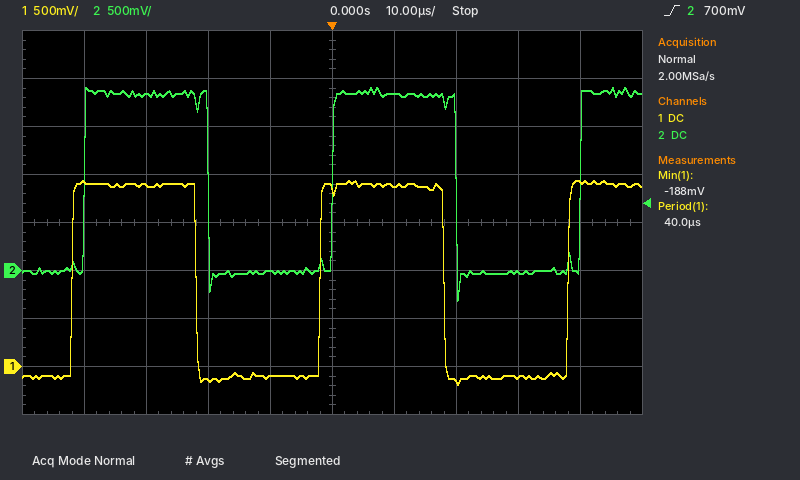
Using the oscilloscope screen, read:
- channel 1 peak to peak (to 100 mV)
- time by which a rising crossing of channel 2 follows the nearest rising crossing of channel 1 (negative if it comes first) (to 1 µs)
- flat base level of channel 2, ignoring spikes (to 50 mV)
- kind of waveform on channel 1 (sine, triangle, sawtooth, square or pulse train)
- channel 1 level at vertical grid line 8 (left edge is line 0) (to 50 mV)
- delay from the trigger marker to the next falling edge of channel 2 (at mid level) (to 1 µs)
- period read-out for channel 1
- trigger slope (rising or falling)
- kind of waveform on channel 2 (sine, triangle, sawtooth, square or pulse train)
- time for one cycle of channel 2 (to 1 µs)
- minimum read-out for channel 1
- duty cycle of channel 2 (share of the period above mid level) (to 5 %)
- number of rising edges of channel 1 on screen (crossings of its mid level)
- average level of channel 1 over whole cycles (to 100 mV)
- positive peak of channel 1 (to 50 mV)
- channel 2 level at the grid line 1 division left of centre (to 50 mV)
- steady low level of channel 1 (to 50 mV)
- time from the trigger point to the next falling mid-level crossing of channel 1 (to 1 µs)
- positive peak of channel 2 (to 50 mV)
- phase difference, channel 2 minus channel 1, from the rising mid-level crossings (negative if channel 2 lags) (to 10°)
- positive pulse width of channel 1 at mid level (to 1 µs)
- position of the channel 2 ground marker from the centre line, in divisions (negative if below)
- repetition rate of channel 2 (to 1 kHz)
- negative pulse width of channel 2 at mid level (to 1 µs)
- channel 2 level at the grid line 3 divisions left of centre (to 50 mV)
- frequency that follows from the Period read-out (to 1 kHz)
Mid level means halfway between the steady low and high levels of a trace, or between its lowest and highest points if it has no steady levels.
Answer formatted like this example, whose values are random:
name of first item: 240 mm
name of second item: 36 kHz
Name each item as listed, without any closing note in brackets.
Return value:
channel 1 peak to peak: 2.10 V
time by which a rising crossing of channel 2 follows the nearest rising crossing of channel 1 (negative if it comes first): +2 µs
flat base level of channel 2, ignoring spikes: 0 mV
kind of waveform on channel 1: square
channel 1 level at vertical grid line 8 (left edge is line 0): -100 mV
delay from the trigger marker to the next falling edge of channel 2 (at mid level): 20 µs
period read-out for channel 1: 40.0 µs
trigger slope: rising
kind of waveform on channel 2: square
time for one cycle of channel 2: 40 µs
minimum read-out for channel 1: -188 mV
duty cycle of channel 2 (share of the period above mid level): 50 %
number of rising edges of channel 1 on screen: 3
average level of channel 1 over whole cycles: 900 mV
positive peak of channel 1: 1.95 V
channel 2 level at the grid line 1 division left of centre: 0 mV
steady low level of channel 1: -100 mV
time from the trigger point to the next falling mid-level crossing of channel 1: 18 µs
positive peak of channel 2: 1.90 V
phase difference, channel 2 minus channel 1, from the rising mid-level crossings (negative if channel 2 lags): -20°
positive pulse width of channel 1 at mid level: 20 µs
position of the channel 2 ground marker from the centre line, in divisions: -1.0 div
repetition rate of channel 2: 25 kHz
negative pulse width of channel 2 at mid level: 20 µs
channel 2 level at the grid line 3 divisions left of centre: 1.85 V
frequency that follows from the Period read-out: 25 kHz
